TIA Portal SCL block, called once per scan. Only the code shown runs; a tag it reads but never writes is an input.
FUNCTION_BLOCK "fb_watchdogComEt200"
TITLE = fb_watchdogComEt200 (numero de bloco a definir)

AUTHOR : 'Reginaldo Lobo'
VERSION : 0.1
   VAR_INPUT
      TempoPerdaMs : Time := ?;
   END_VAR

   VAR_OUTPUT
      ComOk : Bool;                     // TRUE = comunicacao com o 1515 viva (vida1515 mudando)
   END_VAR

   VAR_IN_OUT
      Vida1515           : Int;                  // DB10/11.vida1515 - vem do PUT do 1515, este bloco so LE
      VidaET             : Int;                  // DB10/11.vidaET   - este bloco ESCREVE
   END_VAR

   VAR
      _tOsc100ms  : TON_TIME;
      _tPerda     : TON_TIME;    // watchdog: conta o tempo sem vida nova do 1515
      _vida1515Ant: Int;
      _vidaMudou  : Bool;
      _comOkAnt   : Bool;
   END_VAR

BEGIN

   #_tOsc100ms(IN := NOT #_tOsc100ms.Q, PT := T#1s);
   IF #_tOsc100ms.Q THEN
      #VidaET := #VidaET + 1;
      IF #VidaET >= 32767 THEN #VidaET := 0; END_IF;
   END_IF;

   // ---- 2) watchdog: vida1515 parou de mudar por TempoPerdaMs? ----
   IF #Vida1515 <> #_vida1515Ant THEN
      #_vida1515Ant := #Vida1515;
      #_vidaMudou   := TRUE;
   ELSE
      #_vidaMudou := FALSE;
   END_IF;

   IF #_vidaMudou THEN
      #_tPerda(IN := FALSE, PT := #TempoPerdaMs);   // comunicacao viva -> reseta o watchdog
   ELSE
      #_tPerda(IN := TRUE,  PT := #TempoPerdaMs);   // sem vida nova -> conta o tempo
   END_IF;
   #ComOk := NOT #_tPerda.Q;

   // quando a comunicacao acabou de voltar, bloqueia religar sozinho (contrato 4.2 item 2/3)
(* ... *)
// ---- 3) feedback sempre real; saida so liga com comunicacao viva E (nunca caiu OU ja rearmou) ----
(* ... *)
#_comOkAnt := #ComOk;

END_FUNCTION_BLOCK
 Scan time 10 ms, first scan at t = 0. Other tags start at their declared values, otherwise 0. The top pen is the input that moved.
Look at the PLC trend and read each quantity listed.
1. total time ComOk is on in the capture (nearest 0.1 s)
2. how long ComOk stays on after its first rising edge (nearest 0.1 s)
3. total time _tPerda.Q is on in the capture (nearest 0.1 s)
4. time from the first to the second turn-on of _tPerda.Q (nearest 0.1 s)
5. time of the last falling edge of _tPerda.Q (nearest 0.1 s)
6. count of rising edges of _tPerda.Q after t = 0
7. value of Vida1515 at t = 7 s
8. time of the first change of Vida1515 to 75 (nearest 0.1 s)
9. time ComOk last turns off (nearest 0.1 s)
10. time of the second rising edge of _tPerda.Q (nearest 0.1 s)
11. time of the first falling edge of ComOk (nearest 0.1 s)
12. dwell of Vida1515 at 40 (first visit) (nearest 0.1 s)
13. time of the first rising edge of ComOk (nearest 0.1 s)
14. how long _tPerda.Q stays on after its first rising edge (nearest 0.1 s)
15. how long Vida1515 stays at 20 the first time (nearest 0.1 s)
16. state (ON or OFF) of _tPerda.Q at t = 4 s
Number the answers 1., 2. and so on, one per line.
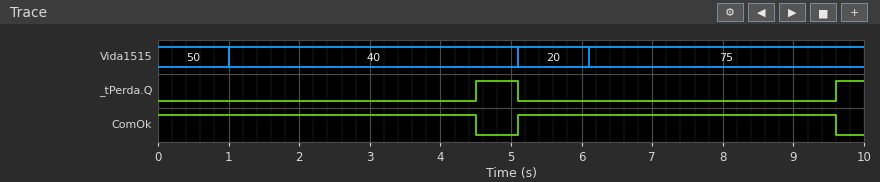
1. 9.0 s
2. 4.5 s
3. 1.0 s
4. 5.1 s
5. 5.1 s
6. 2
7. 75
8. 6.1 s
9. 9.6 s
10. 9.6 s
11. 4.5 s
12. 4.1 s
13. 5.1 s
14. 0.6 s
15. 1.0 s
16. OFF
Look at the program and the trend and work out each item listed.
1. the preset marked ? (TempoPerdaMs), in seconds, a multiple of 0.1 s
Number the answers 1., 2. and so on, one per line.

1. 3.5 s
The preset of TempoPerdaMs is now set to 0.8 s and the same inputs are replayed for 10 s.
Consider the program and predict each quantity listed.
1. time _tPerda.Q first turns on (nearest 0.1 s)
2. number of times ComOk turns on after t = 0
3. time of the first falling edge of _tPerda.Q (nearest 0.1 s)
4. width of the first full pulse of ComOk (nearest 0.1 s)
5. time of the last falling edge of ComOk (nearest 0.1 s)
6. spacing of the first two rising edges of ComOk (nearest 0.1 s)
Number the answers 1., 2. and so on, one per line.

1. 0.8 s
2. 3
3. 1.0 s
4. 0.8 s
5. 6.9 s
6. 4.1 s
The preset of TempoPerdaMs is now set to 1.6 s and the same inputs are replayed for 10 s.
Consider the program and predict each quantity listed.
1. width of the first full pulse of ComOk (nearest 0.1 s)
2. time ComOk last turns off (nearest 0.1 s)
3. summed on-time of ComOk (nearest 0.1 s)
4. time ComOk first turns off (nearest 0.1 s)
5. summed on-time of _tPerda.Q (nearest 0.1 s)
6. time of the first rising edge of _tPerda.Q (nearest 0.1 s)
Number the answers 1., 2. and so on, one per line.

1. 2.6 s
2. 7.7 s
3. 5.2 s
4. 2.6 s
5. 4.8 s
6. 2.6 s
